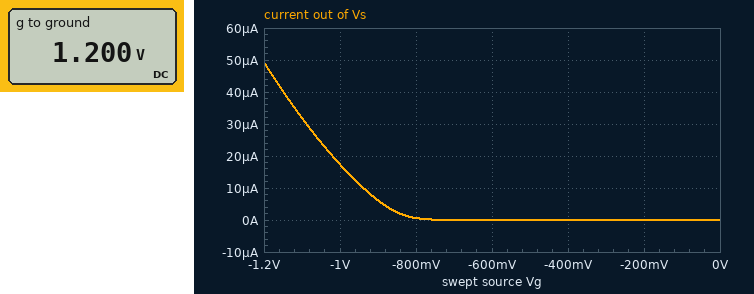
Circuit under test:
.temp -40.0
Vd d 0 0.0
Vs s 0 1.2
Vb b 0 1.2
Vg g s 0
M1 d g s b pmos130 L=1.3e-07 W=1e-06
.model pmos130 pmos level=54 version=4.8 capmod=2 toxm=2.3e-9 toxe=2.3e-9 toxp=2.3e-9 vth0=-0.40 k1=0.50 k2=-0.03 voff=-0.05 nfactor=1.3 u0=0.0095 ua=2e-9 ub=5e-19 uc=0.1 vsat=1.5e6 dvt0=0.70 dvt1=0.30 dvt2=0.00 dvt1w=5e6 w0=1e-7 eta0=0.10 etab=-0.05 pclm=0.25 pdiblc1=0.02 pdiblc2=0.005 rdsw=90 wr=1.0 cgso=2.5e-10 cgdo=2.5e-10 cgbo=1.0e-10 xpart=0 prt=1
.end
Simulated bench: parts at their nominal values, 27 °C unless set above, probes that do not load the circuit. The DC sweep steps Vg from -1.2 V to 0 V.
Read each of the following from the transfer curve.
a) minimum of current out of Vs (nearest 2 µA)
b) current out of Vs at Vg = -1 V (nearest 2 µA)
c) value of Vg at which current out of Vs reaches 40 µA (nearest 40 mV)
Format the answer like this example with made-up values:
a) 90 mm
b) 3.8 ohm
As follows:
a) 0 A
b) 18 µA
c) -1.16 V
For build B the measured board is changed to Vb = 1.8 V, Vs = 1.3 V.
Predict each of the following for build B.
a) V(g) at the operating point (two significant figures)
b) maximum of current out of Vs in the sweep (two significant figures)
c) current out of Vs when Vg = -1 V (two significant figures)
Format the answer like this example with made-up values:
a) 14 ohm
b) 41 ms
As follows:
a) 1.3 V
b) 850 µA
c) 190 µA
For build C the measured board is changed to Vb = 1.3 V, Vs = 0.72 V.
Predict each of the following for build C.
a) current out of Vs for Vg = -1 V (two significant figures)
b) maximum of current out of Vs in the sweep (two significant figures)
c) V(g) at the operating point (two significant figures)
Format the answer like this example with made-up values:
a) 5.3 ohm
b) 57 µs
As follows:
a) 140 µA
b) 740 µA
c) 720 mV
